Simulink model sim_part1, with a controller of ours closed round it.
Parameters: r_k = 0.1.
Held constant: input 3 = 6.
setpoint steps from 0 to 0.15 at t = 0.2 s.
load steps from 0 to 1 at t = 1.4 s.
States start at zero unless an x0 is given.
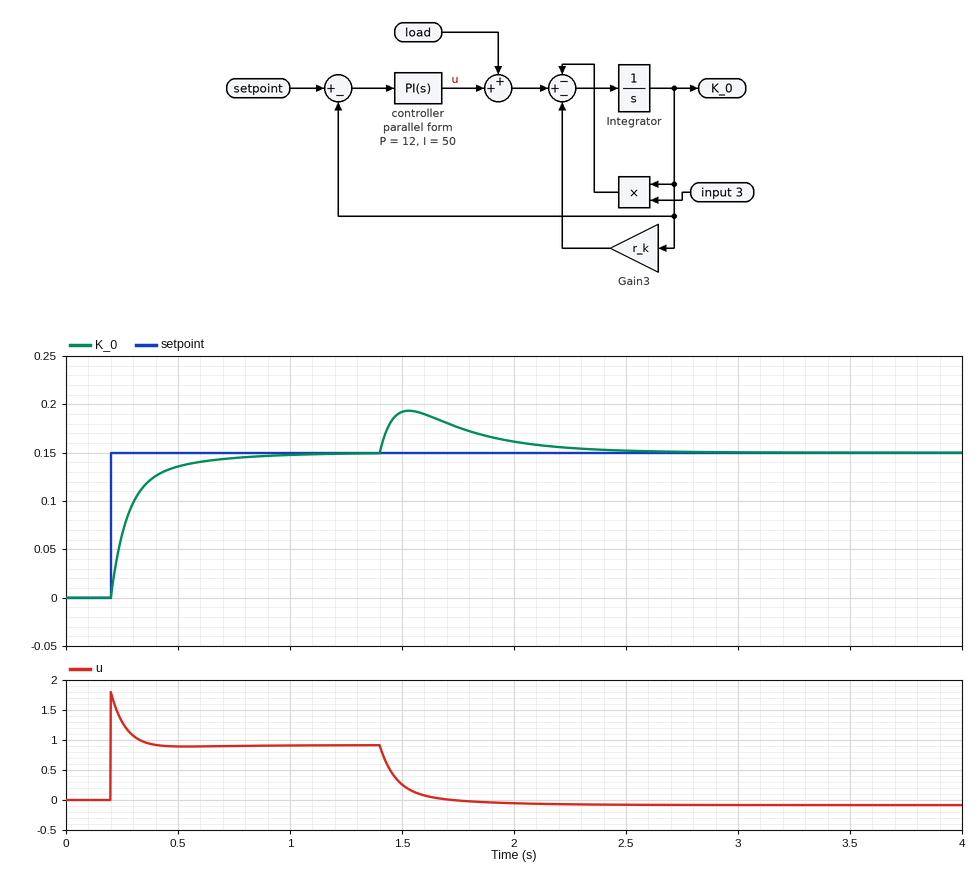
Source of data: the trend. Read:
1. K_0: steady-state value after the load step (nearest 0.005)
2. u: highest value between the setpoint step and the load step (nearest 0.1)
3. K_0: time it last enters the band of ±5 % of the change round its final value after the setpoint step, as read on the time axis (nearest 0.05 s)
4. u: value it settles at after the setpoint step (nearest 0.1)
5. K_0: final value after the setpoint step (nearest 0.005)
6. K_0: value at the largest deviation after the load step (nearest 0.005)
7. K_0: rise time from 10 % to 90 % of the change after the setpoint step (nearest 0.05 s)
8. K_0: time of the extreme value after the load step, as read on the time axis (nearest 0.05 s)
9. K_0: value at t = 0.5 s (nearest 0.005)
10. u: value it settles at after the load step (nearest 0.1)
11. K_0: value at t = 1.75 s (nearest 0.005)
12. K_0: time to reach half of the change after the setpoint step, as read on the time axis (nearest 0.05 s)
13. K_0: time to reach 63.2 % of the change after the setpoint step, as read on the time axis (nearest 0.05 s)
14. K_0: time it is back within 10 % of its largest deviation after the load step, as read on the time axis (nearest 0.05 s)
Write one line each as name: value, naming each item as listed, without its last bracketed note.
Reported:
K_0: steady-state value after the load step: 0.150
u: highest value between the setpoint step and the load step: 1.8
K_0: time it last enters the band of ±5 % of the change round its final value after the setpoint step, as read on the time axis: 0.65 s
u: value it settles at after the setpoint step: 0.9
K_0: final value after the setpoint step: 0.150
K_0: value at the largest deviation after the load step: 0.195
K_0: rise time from 10 % to 90 % of the change after the setpoint step: 0.30 s
K_0: time of the extreme value after the load step, as read on the time axis: 1.55 s
K_0: value at t = 0.5 s: 0.135
u: value it settles at after the load step: -0.1
K_0: value at t = 1.75 s: 0.175
K_0: time to reach half of the change after the setpoint step, as read on the time axis: 0.25 s
K_0: time to reach 63.2 % of the change after the setpoint step, as read on the time axis: 0.30 s
K_0: time it is back within 10 % of its largest deviation after the load step, as read on the time axis: 2.30 s
